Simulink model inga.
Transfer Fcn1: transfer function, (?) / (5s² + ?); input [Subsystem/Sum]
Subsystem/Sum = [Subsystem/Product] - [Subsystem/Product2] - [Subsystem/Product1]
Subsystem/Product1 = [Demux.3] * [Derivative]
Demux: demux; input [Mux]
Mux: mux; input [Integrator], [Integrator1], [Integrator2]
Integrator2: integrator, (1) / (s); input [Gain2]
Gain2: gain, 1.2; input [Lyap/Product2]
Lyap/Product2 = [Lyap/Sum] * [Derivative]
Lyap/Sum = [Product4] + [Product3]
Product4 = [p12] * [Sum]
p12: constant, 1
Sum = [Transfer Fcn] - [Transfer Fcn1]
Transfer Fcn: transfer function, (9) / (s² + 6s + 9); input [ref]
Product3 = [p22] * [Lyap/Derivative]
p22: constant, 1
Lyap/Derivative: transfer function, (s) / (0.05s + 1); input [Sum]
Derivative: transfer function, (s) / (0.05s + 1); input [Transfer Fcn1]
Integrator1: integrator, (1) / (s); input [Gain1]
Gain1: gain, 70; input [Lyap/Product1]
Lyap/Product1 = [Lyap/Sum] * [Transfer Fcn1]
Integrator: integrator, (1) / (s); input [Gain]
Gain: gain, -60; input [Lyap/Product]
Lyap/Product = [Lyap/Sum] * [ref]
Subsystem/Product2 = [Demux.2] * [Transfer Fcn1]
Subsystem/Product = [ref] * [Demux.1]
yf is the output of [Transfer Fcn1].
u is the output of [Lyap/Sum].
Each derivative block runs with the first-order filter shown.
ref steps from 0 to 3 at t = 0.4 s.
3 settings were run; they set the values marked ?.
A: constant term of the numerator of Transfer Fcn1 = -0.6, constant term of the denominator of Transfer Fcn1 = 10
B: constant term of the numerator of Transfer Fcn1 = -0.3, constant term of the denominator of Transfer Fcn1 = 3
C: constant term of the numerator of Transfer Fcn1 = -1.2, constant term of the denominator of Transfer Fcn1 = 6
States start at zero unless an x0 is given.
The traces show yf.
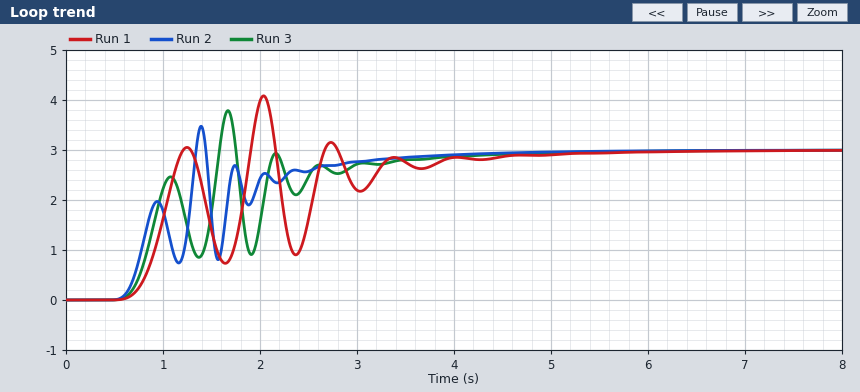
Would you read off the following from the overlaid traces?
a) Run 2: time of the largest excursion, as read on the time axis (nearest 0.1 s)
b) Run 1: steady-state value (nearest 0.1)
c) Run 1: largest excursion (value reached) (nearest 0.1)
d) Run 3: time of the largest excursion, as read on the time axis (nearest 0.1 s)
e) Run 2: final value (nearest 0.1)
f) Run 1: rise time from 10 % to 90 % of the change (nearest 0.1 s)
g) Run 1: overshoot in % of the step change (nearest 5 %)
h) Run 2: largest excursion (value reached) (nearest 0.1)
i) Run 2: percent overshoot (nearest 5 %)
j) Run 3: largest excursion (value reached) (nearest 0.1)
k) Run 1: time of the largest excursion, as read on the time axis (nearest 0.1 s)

1.4 s
3.0
4.1
1.7 s
3.0
0.4 s
35 %
3.5
15 %
3.8
2.0 s
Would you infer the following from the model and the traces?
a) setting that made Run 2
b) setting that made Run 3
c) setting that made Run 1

C
A
B
